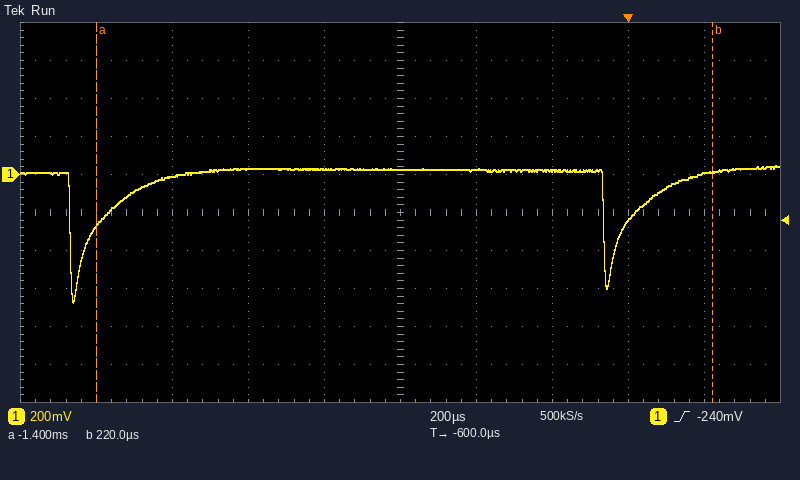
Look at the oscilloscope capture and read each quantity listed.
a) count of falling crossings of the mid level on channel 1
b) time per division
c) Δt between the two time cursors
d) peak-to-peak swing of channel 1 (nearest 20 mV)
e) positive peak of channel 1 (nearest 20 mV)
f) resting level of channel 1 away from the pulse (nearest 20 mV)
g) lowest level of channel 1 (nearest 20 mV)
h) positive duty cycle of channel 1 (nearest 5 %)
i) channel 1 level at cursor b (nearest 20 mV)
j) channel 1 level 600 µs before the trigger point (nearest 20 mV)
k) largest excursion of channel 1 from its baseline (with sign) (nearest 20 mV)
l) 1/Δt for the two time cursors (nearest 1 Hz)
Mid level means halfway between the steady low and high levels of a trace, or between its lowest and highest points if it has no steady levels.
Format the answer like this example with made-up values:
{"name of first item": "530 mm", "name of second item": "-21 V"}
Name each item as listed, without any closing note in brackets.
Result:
{"count of falling crossings of the mid level on channel 1": "2", "time per division": "200 µs", "Δt between the two time cursors": "1.62 ms", "peak-to-peak swing of channel 1": "720 mV", "positive peak of channel 1": "40 mV", "resting level of channel 1 away from the pulse": "20 mV", "lowest level of channel 1": "-680 mV", "positive duty cycle of channel 1": "95 %", "channel 1 level at cursor b": "20 mV", "channel 1 level 600 µs before the trigger point": "20 mV", "largest excursion of channel 1 from its baseline (with sign)": "-700 mV", "1/Δt for the two time cursors": "617 Hz"}
